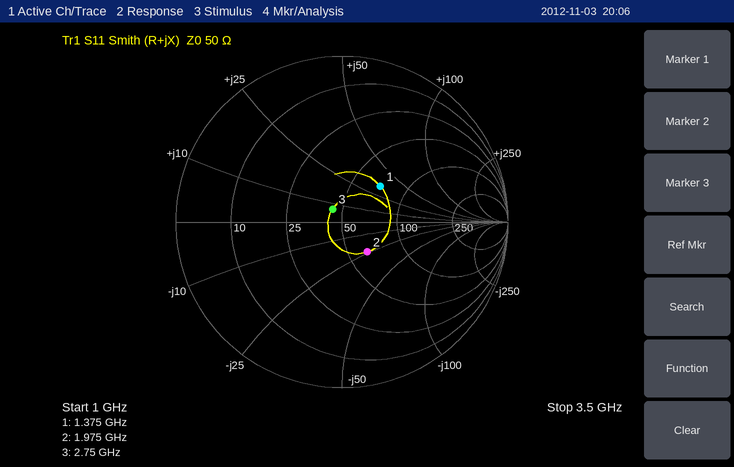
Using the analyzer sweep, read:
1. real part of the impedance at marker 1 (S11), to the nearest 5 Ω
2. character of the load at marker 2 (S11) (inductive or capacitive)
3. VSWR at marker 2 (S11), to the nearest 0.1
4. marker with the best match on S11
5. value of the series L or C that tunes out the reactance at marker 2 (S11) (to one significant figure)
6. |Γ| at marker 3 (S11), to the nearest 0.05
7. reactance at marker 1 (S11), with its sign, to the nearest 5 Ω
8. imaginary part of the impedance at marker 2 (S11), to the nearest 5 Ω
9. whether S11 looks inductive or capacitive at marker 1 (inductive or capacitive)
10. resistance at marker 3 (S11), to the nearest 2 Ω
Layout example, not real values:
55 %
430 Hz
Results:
70 Ω
capacitive
1.6
marker 3
2 nH
0.10
+35 Ω
-25 Ω
inductive
44 Ω
